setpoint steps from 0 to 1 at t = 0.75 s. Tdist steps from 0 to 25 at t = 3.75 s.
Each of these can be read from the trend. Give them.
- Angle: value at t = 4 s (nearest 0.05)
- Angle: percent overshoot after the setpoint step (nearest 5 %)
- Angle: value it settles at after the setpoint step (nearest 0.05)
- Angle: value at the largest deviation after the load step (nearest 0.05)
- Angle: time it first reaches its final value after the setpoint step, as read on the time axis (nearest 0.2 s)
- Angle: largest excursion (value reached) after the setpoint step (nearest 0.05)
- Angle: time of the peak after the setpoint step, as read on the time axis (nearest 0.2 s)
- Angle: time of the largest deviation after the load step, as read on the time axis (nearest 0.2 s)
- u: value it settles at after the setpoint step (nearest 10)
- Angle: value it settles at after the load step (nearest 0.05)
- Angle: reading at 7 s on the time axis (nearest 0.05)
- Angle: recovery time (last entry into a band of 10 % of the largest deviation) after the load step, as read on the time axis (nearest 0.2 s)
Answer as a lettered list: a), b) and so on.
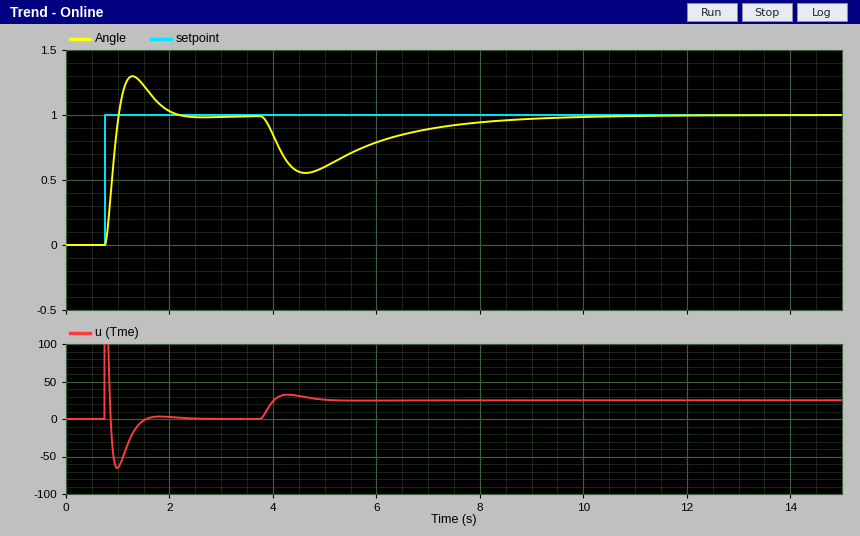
a) 0.85
b) 30 %
c) 1.00
d) 0.55
e) 1.0 s
f) 1.30
g) 1.2 s
h) 4.6 s
i) 0
j) 1.00
k) 0.90
l) 8.4 s
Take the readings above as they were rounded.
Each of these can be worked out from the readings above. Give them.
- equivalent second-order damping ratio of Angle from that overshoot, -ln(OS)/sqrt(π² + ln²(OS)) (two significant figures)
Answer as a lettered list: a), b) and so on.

a) 0.36
